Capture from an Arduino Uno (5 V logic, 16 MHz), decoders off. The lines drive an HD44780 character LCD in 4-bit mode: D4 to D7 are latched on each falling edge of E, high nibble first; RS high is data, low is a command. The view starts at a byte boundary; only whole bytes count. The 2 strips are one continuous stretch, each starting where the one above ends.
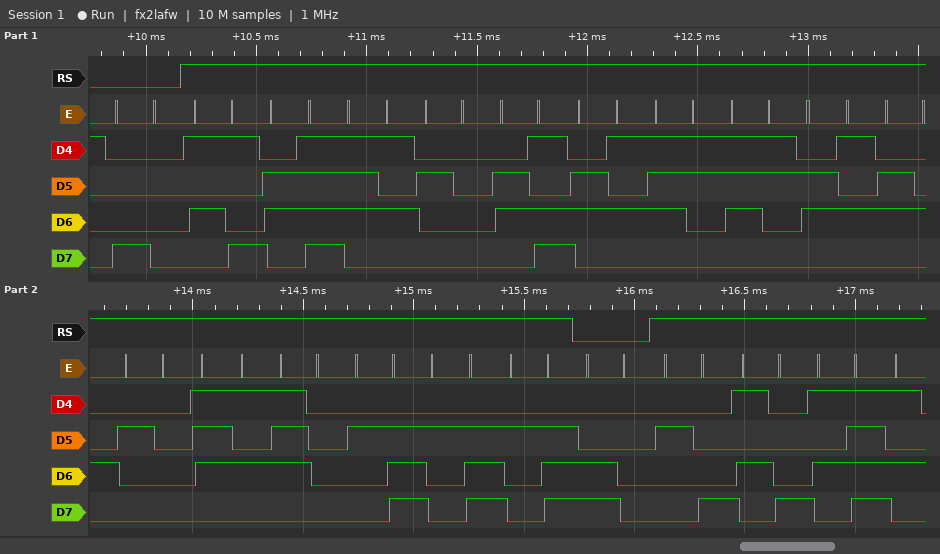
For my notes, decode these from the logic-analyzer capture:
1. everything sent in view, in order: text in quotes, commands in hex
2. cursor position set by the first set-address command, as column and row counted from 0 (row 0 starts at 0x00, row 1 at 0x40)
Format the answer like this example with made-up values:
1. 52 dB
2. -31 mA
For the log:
1. 0x80 "You messed up..." 0xC0 "(X_"
2. column 0, row 0
